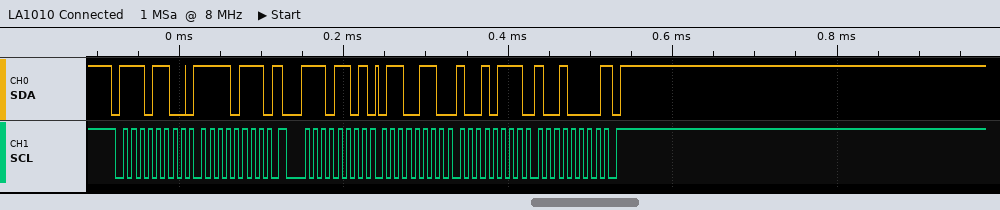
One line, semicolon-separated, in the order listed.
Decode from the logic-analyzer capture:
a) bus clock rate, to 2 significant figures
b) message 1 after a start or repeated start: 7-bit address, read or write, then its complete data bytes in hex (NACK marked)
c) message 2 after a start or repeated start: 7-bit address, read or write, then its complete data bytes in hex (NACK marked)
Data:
100 kHz; 0x76 write: F7; 0x76 read: 66 97 90 NACK
